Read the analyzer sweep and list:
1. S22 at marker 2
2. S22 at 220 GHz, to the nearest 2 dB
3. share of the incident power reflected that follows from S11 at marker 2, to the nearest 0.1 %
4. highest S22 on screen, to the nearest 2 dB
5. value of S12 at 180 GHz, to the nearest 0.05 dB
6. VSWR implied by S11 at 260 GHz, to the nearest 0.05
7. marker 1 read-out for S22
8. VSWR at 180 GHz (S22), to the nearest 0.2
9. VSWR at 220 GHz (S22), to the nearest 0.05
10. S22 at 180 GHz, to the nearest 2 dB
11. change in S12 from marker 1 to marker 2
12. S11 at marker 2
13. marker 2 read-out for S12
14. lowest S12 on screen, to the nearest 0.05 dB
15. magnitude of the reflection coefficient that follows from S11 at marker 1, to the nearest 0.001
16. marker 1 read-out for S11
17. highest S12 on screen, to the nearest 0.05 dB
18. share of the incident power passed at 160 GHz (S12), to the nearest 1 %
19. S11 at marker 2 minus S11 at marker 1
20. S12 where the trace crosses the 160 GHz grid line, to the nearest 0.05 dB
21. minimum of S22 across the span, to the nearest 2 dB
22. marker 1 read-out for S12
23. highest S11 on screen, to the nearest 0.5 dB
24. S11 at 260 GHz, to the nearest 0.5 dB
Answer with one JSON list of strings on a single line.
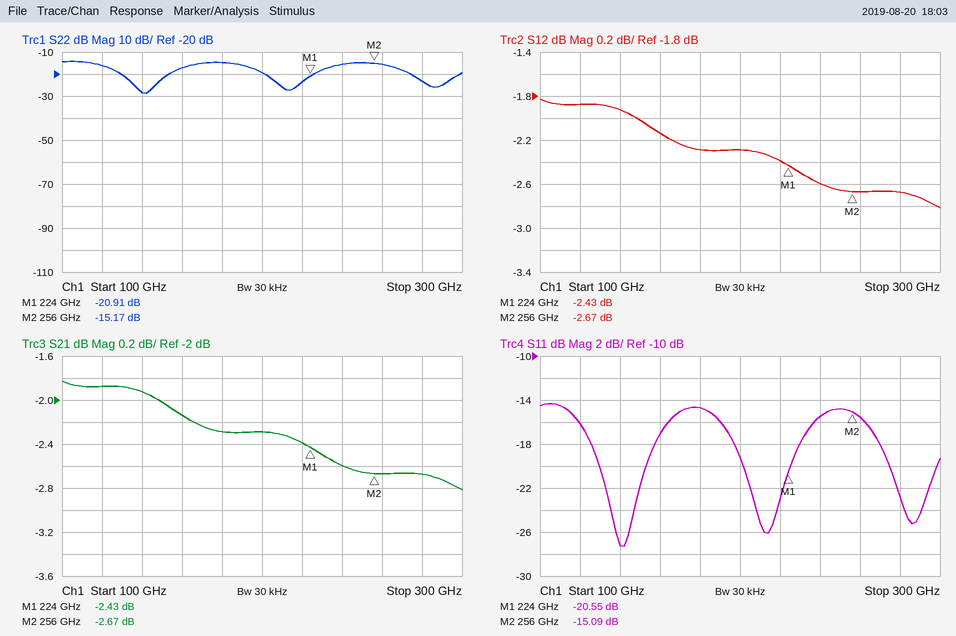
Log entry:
["-15.17 dB", "-24 dB", "3.1 %", "-14 dB", "-2.30 dB", "1.40", "-20.91 dB", "1.4", "1.15", "-14 dB", "-0.24 dB", "-15.09 dB", "-2.67 dB", "-2.80 dB", "0.094", "-20.55 dB", "-1.85 dB", "61 %", "5.46 dB", "-2.15 dB", "-28 dB", "-2.43 dB", "-14.5 dB", "-15.5 dB"]
